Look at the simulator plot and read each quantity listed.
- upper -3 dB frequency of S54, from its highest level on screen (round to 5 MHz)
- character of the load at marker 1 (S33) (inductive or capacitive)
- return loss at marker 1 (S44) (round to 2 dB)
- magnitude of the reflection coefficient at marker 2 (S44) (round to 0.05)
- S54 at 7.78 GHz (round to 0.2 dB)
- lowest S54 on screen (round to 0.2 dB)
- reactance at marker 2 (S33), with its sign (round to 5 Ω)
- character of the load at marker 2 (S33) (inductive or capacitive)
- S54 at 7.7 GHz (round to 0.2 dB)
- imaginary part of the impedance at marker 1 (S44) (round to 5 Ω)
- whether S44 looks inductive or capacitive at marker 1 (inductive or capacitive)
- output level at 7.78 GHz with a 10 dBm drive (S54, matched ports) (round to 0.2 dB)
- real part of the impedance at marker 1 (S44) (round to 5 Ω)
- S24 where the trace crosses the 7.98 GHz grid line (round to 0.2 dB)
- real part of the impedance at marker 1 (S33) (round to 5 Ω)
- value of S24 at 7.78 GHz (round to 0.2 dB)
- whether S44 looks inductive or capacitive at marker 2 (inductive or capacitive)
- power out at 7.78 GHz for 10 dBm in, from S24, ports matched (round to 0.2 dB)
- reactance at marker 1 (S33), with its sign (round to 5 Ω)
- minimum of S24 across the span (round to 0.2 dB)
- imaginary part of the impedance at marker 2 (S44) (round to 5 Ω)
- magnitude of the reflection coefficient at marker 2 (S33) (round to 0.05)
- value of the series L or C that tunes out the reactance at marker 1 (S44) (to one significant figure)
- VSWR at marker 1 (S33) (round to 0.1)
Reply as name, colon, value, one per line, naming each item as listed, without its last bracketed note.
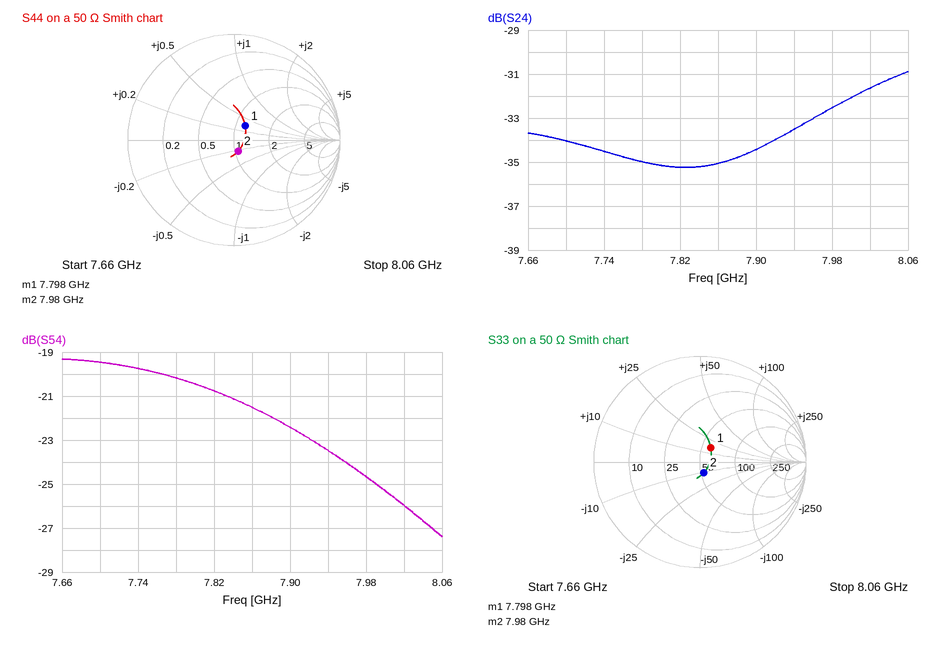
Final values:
upper -3 dB frequency of S54, from its highest level on screen: 7.895 GHz
character of the load at marker 1 (S33): inductive
return loss at marker 1 (S44): 16 dB
magnitude of the reflection coefficient at marker 2 (S44): 0.10
S54 at 7.78 GHz: -20.2 dB
lowest S54 on screen: -27.4 dB
reactance at marker 2 (S33), with its sign: -10 Ω
character of the load at marker 2 (S33): capacitive
S54 at 7.7 GHz: -19.4 dB
imaginary part of the impedance at marker 1 (S44): +15 Ω
whether S44 looks inductive or capacitive at marker 1: inductive
output level at 7.78 GHz with a 10 dBm drive (S54, matched ports): -10.2 dBm
real part of the impedance at marker 1 (S44): 60 Ω
S24 where the trace crosses the 7.98 GHz grid line: -32.6 dB
real part of the impedance at marker 1 (S33): 60 Ω
value of S24 at 7.78 GHz: -35.0 dB
whether S44 looks inductive or capacitive at marker 2: capacitive
power out at 7.78 GHz for 10 dBm in, from S24, ports matched: -25.0 dBm
reactance at marker 1 (S33), with its sign: +15 Ω
minimum of S24 across the span: -35.2 dB
imaginary part of the impedance at marker 2 (S44): -10 Ω
magnitude of the reflection coefficient at marker 2 (S33): 0.10
value of the series L or C that tunes out the reactance at marker 1 (S44): 1 pF
VSWR at marker 1 (S33): 1.4
